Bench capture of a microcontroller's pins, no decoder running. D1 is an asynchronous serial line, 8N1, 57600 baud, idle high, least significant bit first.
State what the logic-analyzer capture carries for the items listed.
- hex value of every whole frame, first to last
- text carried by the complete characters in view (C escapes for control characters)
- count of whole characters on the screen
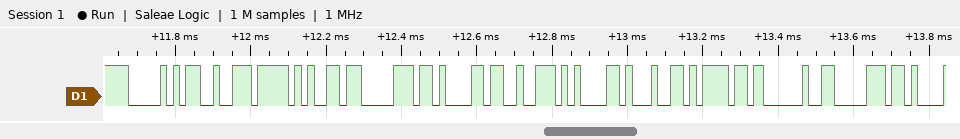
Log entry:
0x50 0x72 0x65 0x70 0x61 0x72 0x61 0x64 0x6F 0x20 0x70
"Preparado p"
11
